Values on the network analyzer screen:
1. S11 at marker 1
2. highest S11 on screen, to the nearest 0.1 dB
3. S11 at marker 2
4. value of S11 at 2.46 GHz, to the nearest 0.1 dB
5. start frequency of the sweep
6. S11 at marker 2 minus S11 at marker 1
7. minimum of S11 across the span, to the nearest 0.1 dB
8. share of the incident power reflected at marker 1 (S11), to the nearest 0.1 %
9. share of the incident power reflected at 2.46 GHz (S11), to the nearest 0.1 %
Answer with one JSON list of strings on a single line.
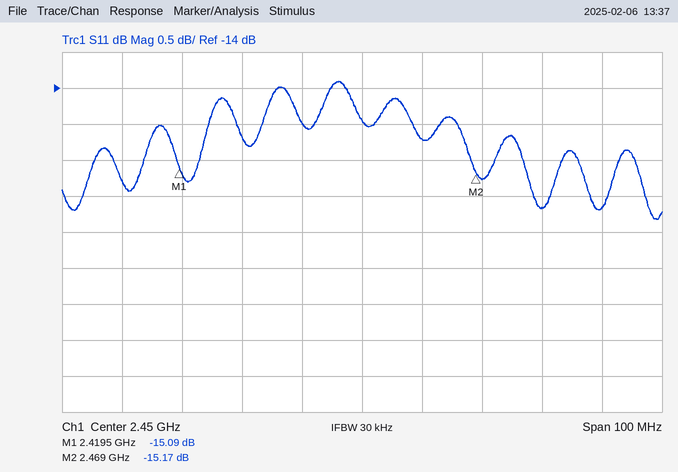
["-15.09 dB", "-13.9 dB", "-15.17 dB", "-14.7 dB", "2.4 GHz", "-0.08 dB", "-15.8 dB", "3.1 %", "3.4 %"]
